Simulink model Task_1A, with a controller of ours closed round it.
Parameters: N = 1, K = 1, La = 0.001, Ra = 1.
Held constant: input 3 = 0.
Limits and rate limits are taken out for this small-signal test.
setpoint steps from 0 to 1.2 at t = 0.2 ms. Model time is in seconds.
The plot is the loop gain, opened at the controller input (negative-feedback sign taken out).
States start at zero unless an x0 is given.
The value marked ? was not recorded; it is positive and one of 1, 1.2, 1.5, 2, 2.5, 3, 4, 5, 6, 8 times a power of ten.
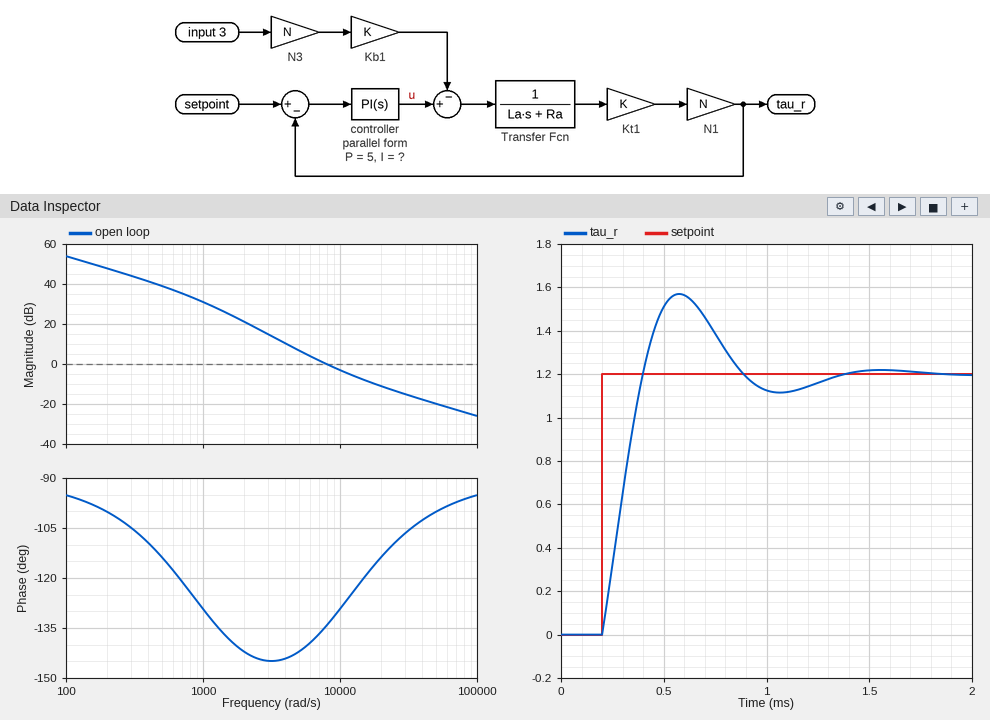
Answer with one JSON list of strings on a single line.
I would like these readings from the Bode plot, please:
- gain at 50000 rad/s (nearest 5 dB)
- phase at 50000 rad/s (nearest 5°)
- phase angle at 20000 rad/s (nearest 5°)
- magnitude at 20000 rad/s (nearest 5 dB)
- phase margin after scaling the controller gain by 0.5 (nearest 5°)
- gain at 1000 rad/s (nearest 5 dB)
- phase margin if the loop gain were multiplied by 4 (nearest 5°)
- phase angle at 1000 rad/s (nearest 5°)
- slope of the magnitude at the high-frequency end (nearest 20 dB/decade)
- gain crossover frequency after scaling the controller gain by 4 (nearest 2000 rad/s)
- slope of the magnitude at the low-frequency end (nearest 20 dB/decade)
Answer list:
["-20 dB", "-100°", "-115°", "-10 dB", "40°", "30 dB", "70°", "-130°", "-20 dB/decade", "22000 rad/s", "-20 dB/decade"]
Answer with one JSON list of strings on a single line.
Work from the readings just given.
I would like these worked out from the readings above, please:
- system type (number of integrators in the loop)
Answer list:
["1"]
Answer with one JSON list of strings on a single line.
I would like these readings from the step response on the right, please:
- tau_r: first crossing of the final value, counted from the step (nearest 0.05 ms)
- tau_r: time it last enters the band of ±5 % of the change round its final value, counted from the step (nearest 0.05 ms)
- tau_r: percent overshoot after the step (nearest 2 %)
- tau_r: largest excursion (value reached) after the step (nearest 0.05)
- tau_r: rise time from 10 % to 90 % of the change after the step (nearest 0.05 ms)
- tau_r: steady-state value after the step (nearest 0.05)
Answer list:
["0.20 ms", "1.00 ms", "30 %", "1.55", "0.15 ms", "1.20"]
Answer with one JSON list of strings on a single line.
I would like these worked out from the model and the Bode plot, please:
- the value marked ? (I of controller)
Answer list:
["50000"]
